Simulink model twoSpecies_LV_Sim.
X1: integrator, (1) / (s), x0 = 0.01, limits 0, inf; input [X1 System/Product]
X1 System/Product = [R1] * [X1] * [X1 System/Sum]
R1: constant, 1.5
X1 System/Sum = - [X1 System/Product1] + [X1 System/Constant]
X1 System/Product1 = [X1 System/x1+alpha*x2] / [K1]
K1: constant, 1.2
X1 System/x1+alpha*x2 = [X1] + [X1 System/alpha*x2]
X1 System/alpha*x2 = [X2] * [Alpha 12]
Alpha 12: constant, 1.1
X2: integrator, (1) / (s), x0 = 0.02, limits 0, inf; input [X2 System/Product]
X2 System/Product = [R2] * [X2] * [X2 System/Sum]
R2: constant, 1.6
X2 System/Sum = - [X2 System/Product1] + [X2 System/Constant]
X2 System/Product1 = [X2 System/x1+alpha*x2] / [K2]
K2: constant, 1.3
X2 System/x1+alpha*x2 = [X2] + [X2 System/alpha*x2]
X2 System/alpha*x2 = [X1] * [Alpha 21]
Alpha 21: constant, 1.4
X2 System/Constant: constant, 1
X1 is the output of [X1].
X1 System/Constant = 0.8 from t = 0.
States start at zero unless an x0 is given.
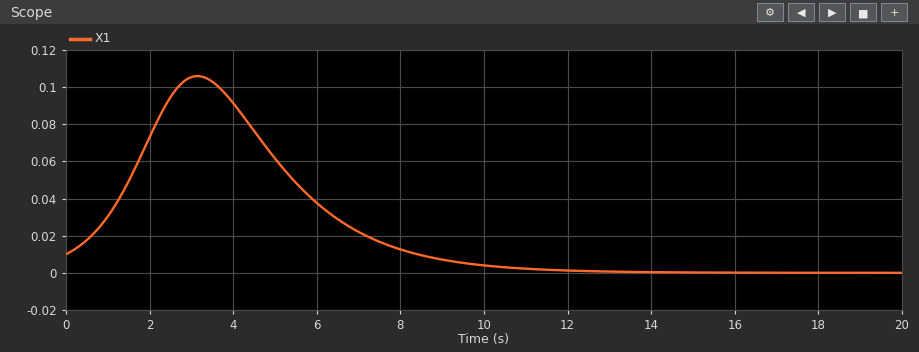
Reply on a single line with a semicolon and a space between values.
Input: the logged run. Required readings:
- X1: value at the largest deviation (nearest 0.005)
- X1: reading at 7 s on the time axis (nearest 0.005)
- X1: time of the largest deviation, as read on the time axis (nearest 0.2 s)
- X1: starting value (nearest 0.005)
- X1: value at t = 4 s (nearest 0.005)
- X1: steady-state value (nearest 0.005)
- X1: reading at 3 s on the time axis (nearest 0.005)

0.105; 0.020; 3.2 s; 0.010; 0.090; 0.000; 0.105
